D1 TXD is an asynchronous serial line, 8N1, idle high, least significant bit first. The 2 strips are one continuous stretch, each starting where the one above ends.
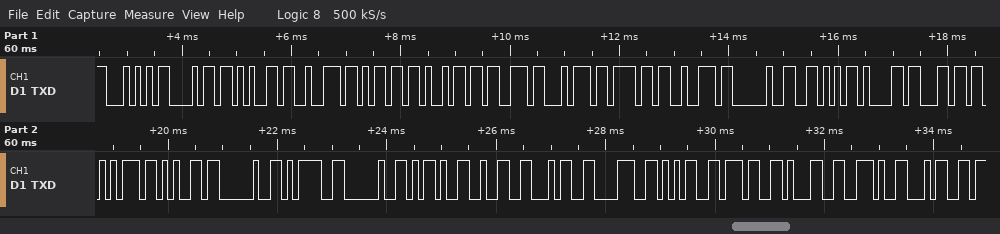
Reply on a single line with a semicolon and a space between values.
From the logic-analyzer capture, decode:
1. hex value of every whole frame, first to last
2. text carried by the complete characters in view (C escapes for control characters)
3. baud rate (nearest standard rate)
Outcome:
0x54 0x68 0x65 0x72 0x6D 0x69 0x73 0x74 0x6F 0x72 0x20 0x56 0x61 0x6C 0x75 0x65 0x20 0x3D 0x20 0x2D 0x32 0x34 0x38 0x35 0x37 0x31 0x2E 0x34; "Thermistor Value = -248571.4"; 9600 baud
